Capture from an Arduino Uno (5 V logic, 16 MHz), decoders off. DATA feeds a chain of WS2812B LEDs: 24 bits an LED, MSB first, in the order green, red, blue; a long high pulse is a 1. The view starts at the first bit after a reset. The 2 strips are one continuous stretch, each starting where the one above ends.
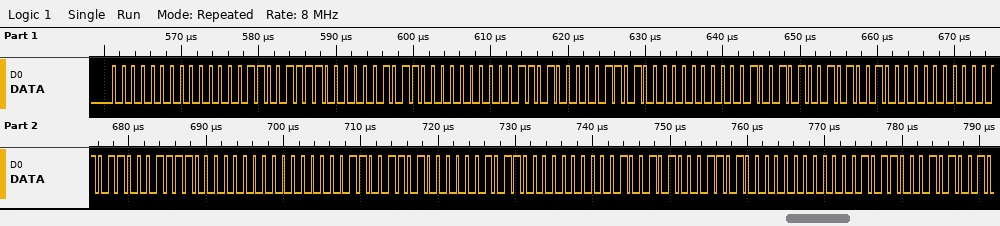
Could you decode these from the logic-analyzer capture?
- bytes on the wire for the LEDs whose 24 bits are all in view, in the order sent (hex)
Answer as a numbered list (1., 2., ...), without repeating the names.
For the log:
1. 00 03 3C 0B 00 34 1A 00 25 29 00 16 3C 00 03 34 0B 00 25 1A 00
